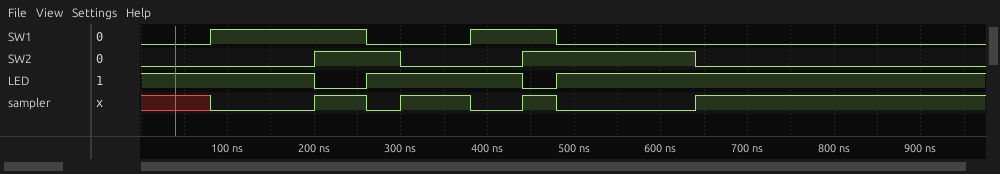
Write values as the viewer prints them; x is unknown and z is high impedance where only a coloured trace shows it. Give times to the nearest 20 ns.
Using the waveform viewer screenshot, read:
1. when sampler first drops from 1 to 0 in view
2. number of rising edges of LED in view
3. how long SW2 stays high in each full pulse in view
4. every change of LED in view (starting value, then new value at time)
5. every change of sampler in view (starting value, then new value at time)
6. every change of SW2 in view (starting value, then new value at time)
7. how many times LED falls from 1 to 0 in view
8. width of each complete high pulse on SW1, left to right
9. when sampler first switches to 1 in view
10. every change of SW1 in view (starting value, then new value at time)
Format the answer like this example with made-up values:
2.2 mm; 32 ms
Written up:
260 ns; 2; 100 ns, 200 ns; 1, 0 at 200 ns, 1 at 260 ns, 0 at 440 ns, 1 at 480 ns; x, 0 at 80 ns, 1 at 200 ns, 0 at 260 ns, 1 at 300 ns, 0 at 380 ns, 1 at 440 ns, 0 at 480 ns, 1 at 640 ns; 0, 1 at 200 ns, 0 at 300 ns, 1 at 440 ns, 0 at 640 ns; 2; 180 ns, 100 ns; 200 ns; 0, 1 at 80 ns, 0 at 260 ns, 1 at 380 ns, 0 at 480 ns
